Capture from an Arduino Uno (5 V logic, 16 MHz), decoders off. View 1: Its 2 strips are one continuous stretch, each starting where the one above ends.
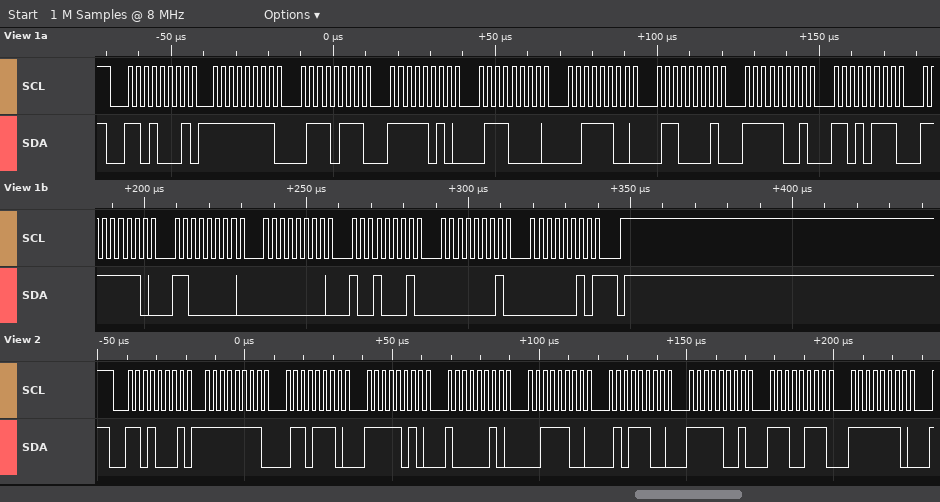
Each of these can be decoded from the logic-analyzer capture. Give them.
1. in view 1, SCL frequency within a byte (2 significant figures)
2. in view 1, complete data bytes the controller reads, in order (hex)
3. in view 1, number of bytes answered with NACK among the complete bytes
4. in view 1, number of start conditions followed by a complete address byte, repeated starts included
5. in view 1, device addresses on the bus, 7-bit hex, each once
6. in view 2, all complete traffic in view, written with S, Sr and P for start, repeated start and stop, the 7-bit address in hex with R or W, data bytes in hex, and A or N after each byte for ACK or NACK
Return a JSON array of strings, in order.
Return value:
["400 kHz", "FF 77 FA 70 3C 61 F9 D7 FE C0 00 91 01 02", "1", "1", "0x68", "S 68R A FF A 6E A FA A 82 A 3C A 5C A F9 A E7 A FE A"]
